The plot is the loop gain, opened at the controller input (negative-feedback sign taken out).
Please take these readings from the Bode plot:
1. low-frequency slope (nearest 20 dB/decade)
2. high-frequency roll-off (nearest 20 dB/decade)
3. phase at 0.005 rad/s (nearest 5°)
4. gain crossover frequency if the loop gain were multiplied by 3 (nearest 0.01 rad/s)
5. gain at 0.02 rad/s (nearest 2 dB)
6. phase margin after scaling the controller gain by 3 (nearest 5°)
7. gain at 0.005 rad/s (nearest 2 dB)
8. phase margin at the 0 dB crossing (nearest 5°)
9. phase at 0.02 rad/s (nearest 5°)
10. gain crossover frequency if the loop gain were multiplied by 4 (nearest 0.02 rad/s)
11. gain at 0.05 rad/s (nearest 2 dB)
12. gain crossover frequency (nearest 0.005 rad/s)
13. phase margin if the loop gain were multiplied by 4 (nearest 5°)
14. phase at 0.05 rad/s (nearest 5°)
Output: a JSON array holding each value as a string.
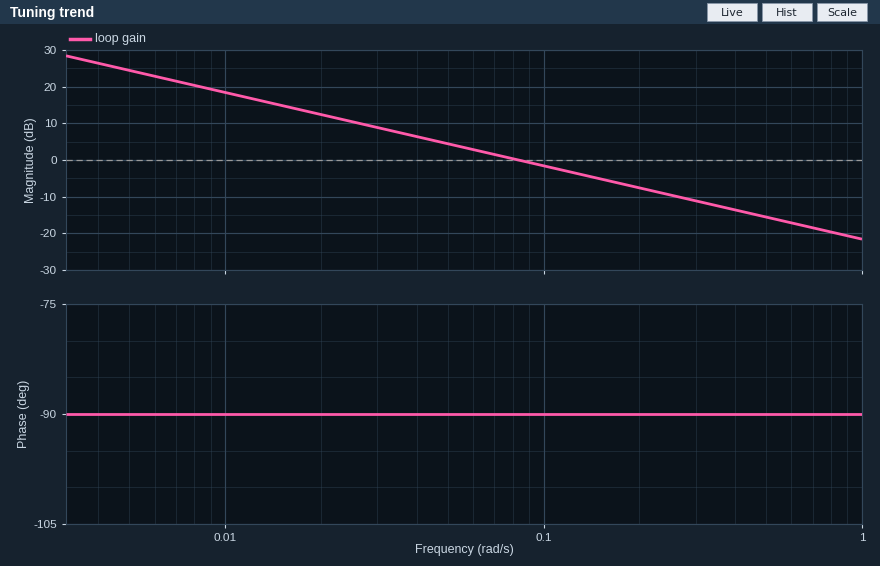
["-20 dB/decade", "-20 dB/decade", "-90°", "0.25 rad/s", "12 dB", "90°", "24 dB", "90°", "-90°", "0.34 rad/s", "4 dB", "0.085 rad/s", "90°", "-90°"]
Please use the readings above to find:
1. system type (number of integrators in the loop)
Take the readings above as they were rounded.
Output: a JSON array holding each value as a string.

["1"]
